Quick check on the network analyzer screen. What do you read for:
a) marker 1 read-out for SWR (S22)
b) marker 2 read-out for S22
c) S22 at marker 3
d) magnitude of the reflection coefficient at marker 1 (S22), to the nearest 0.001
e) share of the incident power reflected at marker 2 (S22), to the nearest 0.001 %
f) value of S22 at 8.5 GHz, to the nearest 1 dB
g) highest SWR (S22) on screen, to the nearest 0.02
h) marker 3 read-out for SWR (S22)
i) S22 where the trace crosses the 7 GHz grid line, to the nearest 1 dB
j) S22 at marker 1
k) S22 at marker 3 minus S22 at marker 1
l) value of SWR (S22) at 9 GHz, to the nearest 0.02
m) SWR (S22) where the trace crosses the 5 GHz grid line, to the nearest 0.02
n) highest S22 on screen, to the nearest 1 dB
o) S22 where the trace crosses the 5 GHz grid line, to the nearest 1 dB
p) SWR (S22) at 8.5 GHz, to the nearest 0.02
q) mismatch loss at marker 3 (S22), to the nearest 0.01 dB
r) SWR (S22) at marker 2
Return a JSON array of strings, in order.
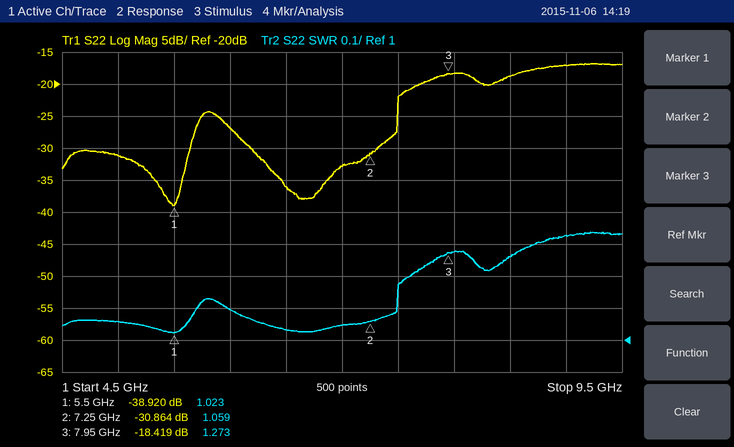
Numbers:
["1.023", "-30.864 dB", "-18.419 dB", "0.011", "0.082 %", "-19 dB", "1.34", "1.273", "-33 dB", "-38.920 dB", "20.501 dB", "1.32", "1.06", "-17 dB", "-31 dB", "1.26", "0.06 dB", "1.059"]
